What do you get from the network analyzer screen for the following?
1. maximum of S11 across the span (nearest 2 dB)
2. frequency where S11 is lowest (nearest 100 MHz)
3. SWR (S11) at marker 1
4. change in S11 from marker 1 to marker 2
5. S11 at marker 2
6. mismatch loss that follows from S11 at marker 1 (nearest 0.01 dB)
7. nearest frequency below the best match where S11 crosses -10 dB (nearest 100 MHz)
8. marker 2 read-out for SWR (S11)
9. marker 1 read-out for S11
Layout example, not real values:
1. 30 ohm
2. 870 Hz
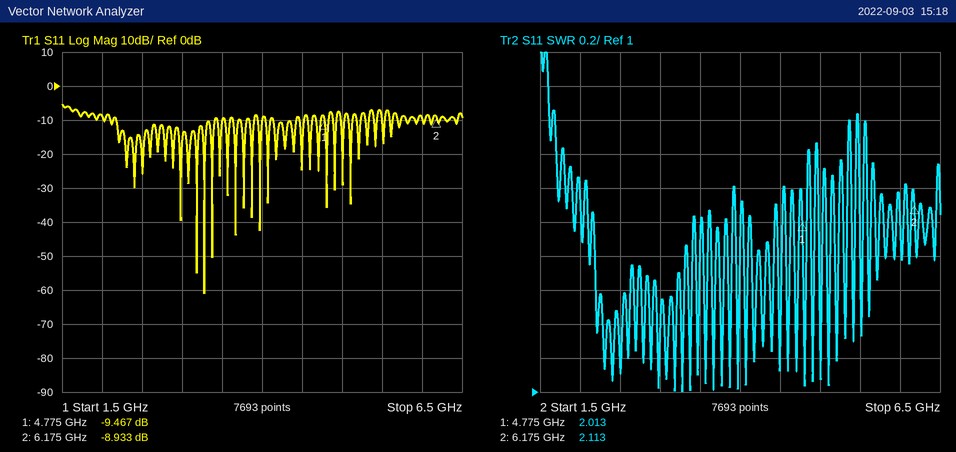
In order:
1. -6 dB
2. 3.3 GHz
3. 2.013
4. 0.534 dB
5. -8.933 dB
6. 0.52 dB
7. 2.2 GHz
8. 2.113
9. -9.467 dB
